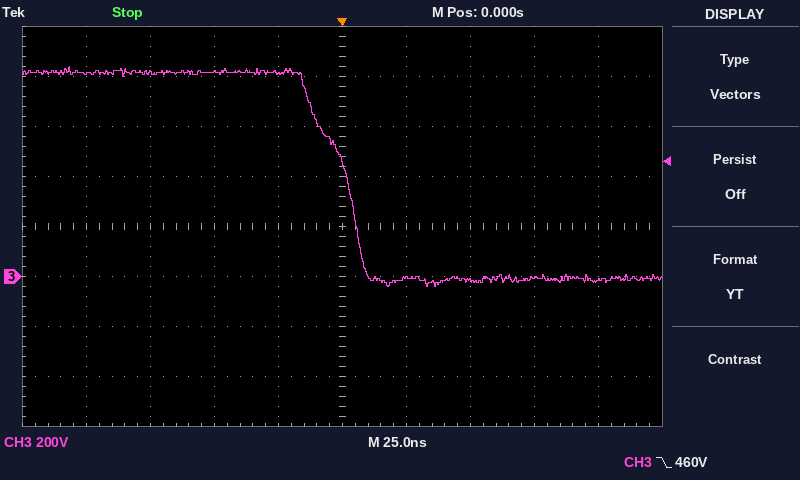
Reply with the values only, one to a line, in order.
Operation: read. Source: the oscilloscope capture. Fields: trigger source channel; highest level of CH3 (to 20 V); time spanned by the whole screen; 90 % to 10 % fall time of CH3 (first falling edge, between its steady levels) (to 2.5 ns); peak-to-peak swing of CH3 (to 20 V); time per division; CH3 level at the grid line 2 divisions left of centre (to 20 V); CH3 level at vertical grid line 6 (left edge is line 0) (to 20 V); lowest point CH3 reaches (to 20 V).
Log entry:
CH3
840 V
250 ns
22.5 ns
880 V
25 ns
820 V
0 V
-40 V
